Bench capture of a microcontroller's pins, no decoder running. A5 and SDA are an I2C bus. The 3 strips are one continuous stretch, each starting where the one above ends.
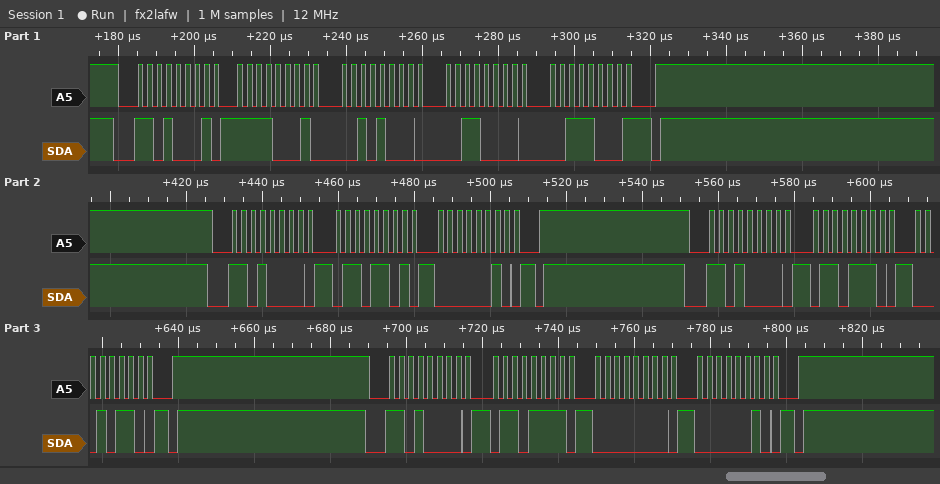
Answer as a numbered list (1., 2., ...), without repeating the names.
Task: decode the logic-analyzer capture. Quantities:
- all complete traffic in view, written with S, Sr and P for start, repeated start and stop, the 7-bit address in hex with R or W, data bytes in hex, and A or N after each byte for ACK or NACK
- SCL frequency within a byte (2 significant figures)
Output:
1. S 68R A F1 A 28 A 30 A 38 N P S 68W A 6D A 02 A P S 68W A 6E A 16 A P S 68W A 6F A 00 A 02 A P
2. 400 kHz
